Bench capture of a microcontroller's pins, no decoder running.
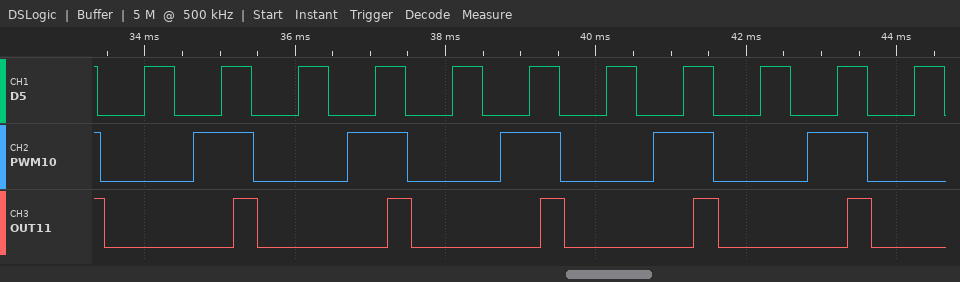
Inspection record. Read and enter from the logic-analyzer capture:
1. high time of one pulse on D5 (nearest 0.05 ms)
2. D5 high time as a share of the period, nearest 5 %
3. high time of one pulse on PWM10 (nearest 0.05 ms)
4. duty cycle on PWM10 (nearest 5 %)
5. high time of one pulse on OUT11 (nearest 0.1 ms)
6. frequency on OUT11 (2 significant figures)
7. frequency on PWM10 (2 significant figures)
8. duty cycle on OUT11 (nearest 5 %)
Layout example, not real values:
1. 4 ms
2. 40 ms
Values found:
1. 0.40 ms
2. 40 %
3. 0.80 ms
4. 40 %
5. 0.3 ms
6. 490 Hz
7. 490 Hz
8. 15 %
